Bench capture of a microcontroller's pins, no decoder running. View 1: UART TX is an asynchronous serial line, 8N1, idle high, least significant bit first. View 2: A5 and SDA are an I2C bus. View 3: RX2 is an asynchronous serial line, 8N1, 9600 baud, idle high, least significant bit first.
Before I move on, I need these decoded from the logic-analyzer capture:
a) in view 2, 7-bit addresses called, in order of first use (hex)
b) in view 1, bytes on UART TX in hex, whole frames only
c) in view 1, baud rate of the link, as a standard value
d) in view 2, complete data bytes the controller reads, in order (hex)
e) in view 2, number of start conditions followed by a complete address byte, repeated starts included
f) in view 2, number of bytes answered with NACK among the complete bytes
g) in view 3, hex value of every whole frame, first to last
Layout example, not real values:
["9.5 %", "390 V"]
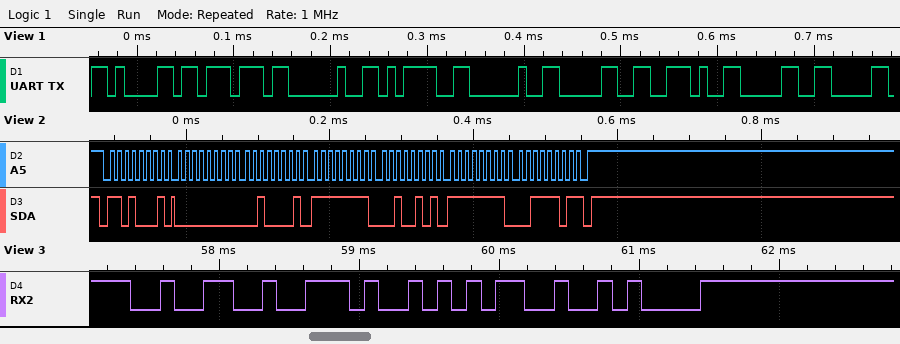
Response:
["0x68", "61 77 20 3D 20 30 2E 30", "115200 baud", "00 21 FF 25 FF 3D", "1", "1", "0x32 0x2E 0x35 0x0A"]
